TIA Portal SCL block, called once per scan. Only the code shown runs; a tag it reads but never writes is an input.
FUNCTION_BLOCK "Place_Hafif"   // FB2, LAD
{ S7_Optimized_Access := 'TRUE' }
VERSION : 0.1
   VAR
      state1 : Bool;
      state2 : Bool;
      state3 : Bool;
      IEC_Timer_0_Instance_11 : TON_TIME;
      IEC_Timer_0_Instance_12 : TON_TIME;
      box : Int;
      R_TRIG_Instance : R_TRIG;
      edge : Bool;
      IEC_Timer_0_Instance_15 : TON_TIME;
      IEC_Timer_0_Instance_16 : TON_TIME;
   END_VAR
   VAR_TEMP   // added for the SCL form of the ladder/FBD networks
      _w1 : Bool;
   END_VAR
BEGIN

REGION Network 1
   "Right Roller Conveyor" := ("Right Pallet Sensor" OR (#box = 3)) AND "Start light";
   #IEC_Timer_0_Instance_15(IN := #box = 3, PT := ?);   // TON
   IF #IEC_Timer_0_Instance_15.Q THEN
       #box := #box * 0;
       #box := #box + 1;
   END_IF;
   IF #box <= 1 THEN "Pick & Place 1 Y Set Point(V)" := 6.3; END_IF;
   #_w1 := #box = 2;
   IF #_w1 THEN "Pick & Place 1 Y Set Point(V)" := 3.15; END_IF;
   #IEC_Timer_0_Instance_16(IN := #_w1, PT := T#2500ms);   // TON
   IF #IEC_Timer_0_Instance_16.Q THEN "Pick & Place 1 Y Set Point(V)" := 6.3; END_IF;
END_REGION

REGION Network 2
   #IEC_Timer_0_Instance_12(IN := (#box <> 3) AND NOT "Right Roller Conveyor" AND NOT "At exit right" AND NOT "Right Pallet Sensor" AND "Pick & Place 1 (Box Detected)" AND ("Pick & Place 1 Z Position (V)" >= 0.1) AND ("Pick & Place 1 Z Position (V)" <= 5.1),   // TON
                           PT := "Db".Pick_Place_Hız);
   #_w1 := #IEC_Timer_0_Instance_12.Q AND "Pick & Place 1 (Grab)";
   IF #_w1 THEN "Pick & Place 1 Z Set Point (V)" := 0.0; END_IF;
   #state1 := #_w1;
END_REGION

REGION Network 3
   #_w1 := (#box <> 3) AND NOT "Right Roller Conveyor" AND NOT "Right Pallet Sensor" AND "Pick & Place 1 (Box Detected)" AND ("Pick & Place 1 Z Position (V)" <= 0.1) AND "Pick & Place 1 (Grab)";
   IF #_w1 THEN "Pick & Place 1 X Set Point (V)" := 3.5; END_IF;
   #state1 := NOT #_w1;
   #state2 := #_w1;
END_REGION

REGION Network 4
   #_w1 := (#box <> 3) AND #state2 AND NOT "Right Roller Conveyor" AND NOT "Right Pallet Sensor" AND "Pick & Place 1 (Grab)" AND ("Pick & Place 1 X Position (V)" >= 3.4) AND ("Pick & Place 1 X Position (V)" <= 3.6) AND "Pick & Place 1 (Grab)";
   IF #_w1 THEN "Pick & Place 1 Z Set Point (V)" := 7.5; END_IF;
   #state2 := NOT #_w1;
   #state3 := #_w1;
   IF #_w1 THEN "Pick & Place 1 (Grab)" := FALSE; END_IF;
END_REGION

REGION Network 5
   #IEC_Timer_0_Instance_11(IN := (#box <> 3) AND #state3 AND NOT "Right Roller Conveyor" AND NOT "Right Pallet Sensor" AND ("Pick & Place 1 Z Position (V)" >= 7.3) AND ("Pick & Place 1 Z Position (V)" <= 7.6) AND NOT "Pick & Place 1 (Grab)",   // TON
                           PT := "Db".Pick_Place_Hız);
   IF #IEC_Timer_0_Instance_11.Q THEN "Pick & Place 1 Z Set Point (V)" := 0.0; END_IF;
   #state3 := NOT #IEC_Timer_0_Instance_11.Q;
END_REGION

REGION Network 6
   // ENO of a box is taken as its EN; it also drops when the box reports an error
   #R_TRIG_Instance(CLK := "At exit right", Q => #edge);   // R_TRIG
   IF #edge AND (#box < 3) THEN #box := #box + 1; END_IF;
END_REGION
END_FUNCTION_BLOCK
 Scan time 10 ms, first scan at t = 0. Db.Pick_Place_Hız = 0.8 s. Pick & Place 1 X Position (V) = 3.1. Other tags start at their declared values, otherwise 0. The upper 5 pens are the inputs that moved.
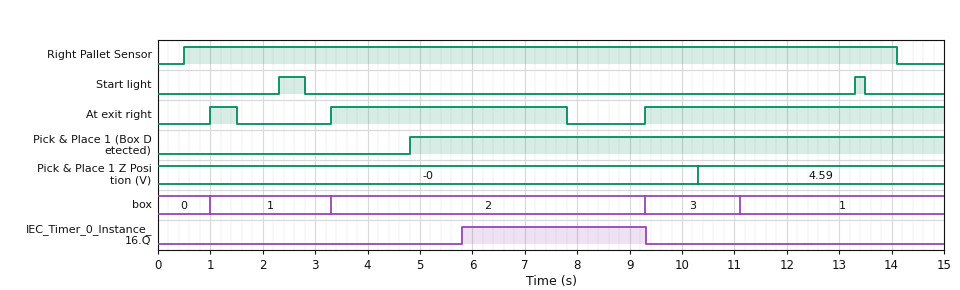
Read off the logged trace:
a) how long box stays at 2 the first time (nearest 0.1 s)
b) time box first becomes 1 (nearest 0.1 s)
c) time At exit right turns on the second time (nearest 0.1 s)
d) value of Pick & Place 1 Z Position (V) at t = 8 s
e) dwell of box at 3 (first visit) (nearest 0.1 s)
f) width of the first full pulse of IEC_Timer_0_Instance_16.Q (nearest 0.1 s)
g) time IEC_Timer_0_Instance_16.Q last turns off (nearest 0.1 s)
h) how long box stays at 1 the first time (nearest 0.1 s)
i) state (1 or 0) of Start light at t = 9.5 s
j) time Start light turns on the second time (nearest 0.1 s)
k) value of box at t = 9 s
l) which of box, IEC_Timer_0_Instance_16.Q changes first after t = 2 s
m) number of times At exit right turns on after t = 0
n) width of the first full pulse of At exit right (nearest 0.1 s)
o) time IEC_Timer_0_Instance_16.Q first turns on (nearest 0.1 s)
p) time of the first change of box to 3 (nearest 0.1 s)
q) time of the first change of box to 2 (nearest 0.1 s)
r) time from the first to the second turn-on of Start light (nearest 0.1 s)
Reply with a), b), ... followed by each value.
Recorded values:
a) 6.0 s
b) 1.0 s
c) 3.3 s
d) -0
e) 1.8 s
f) 3.5 s
g) 9.3 s
h) 2.3 s
i) 0
j) 13.3 s
k) 2
l) box
m) 3
n) 0.5 s
o) 5.8 s
p) 9.3 s
q) 3.3 s
r) 11.0 s
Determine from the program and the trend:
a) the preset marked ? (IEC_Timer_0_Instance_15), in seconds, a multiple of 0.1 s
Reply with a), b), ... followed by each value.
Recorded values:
a) 1.8 s
